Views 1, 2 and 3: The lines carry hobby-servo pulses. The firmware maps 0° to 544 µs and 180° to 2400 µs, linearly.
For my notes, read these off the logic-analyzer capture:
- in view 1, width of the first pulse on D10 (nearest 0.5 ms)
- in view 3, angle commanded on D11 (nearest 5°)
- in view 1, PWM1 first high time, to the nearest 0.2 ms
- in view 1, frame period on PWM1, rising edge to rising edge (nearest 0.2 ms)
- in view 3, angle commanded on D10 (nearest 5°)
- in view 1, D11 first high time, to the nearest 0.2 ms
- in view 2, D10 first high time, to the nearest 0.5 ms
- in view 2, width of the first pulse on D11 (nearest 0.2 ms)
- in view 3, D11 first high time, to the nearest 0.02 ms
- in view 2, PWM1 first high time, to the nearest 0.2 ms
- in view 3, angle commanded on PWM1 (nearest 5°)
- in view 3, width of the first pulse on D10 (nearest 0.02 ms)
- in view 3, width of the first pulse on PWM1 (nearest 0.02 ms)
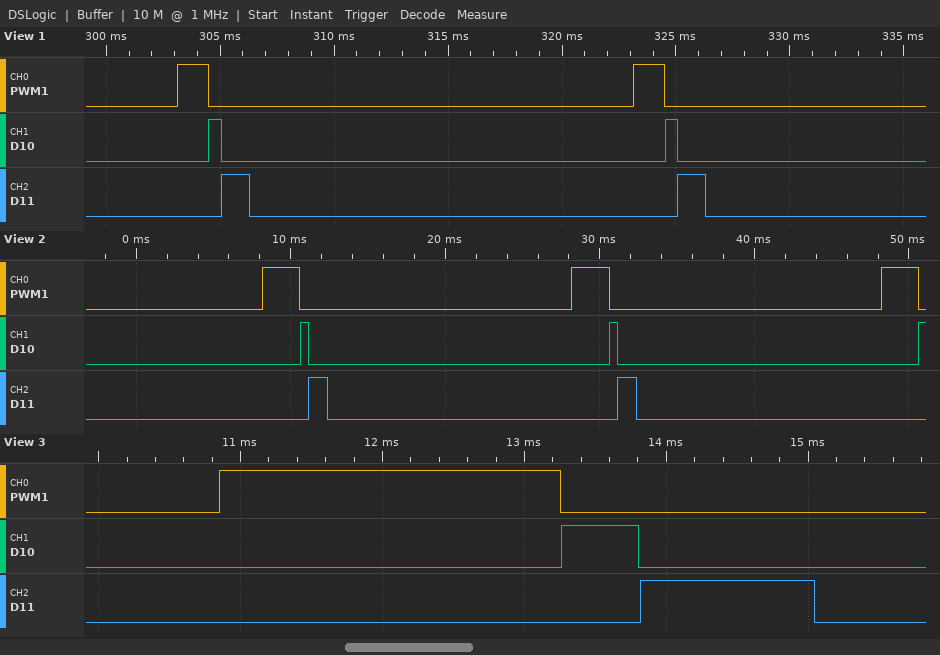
0.5 ms
65°
1.4 ms
20.0 ms
0°
1.2 ms
0.5 ms
1.2 ms
1.22 ms
2.4 ms
180°
0.54 ms
2.40 ms
